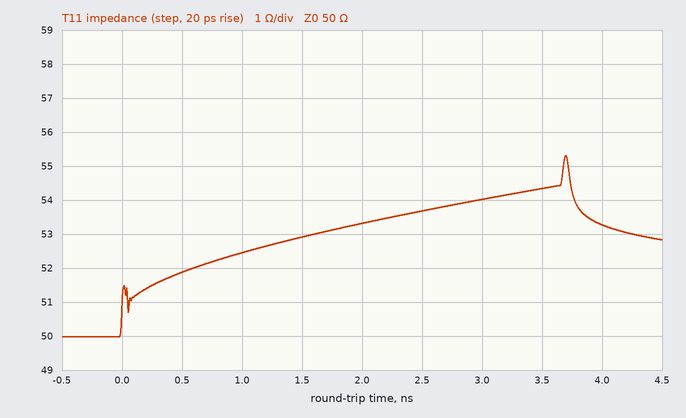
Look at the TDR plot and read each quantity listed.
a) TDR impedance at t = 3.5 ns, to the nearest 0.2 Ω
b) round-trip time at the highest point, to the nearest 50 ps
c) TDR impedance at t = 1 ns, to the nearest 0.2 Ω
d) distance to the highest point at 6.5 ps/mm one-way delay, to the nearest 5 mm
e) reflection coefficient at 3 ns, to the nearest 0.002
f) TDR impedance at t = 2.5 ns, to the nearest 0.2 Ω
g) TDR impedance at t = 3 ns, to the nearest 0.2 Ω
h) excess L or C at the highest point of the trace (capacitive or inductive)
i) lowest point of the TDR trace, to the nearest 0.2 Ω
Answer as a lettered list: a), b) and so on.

a) 54.4 Ω
b) 3.70 ns
c) 52.4 Ω
d) 285 mm
e) +0.038
f) 53.6 Ω
g) 54.0 Ω
h) inductive
i) 50.0 Ω
